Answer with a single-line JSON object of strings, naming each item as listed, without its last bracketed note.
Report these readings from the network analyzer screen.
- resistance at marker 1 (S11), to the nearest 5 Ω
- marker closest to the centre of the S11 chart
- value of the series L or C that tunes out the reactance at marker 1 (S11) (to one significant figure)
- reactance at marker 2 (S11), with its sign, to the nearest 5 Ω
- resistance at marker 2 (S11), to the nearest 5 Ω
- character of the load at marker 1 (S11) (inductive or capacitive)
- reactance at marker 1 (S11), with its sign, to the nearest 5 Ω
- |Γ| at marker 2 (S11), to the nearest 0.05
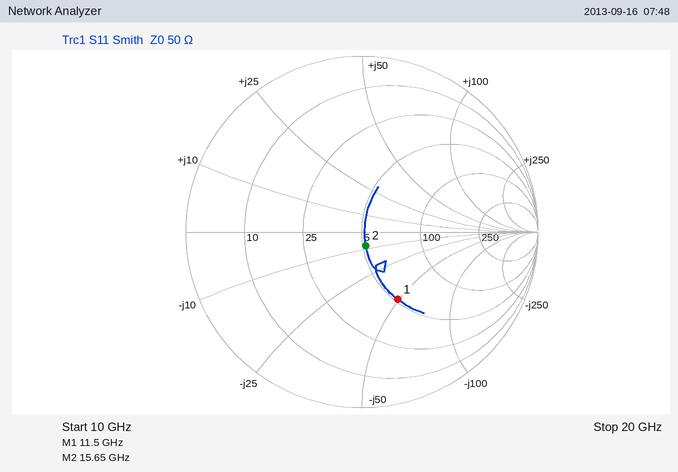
{"resistance at marker 1 (S11), to the nearest 5 Ω": "50 Ω", "marker closest to the centre of the S11 chart": "marker 2", "value of the series L or C that tunes out the reactance at marker 1 (S11)": "700 pH", "reactance at marker 2 (S11), with its sign, to the nearest 5 Ω": "-10 Ω", "resistance at marker 2 (S11), to the nearest 5 Ω": "50 Ω", "character of the load at marker 1 (S11)": "capacitive", "reactance at marker 1 (S11), with its sign, to the nearest 5 Ω": "-50 Ω", "|Γ| at marker 2 (S11), to the nearest 0.05": "0.10"}
